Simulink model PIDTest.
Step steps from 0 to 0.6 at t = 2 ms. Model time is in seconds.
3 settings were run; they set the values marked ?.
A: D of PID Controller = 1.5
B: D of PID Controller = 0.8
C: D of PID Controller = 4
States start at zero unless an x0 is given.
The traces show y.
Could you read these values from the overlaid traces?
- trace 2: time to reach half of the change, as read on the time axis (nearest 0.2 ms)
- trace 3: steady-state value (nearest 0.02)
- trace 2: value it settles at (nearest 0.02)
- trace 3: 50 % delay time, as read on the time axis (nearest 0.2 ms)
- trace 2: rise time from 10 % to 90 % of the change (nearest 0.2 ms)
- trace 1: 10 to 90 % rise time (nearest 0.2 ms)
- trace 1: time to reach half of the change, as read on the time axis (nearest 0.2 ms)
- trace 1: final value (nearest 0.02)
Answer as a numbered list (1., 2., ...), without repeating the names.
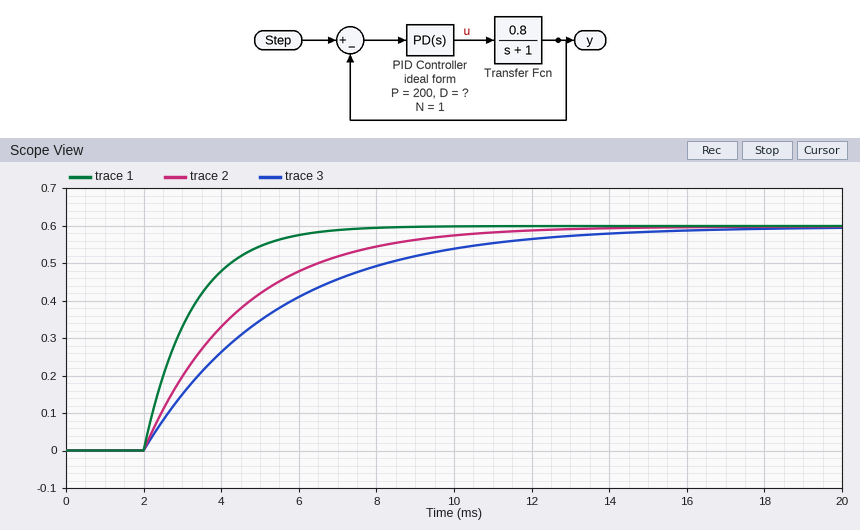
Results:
1. 3.8 ms
2. 0.60
3. 0.60
4. 4.4 ms
5. 5.4 ms
6. 2.8 ms
7. 2.8 ms
8. 0.60
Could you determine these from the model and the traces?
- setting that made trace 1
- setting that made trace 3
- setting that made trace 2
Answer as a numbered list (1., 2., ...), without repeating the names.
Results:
1. C
2. B
3. A
